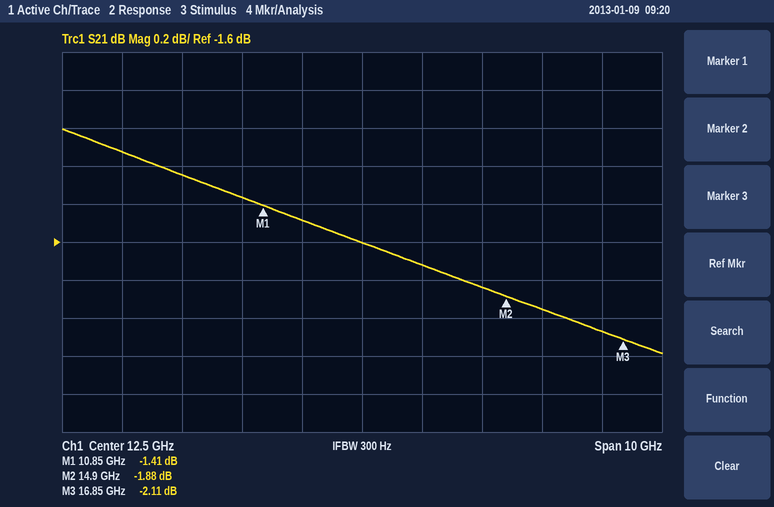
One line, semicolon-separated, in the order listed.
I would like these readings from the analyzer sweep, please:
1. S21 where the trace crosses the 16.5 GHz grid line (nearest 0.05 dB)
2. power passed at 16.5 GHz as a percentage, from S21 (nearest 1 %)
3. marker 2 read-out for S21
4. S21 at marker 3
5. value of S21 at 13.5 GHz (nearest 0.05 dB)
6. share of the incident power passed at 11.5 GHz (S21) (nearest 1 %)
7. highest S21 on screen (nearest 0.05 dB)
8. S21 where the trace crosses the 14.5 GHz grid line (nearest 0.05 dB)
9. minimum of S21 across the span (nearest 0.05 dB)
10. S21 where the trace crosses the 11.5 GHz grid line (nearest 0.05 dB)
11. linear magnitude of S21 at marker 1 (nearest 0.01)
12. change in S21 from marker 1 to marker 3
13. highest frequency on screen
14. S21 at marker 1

-2.05 dB; 62 %; -1.88 dB; -2.11 dB; -1.70 dB; 71 %; -1.00 dB; -1.85 dB; -2.20 dB; -1.50 dB; 0.85; -0.70 dB; 17.5 GHz; -1.41 dB
